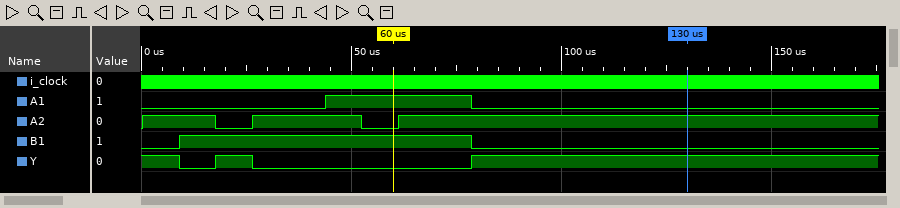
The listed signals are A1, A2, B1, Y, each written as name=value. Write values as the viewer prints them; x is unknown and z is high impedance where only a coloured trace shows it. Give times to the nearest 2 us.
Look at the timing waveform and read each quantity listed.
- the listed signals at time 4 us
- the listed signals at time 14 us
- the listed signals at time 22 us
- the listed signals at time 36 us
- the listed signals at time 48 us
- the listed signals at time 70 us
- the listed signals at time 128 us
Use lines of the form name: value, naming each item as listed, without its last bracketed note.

the listed signals at time 4 us: A1=0, A2=1, B1=0, Y=1
the listed signals at time 14 us: A1=0, A2=1, B1=1, Y=0
the listed signals at time 22 us: A1=0, A2=0, B1=1, Y=1
the listed signals at time 36 us: A1=0, A2=1, B1=1, Y=0
the listed signals at time 48 us: A1=1, A2=1, B1=1, Y=0
the listed signals at time 70 us: A1=1, A2=1, B1=1, Y=0
the listed signals at time 128 us: A1=0, A2=1, B1=0, Y=1
